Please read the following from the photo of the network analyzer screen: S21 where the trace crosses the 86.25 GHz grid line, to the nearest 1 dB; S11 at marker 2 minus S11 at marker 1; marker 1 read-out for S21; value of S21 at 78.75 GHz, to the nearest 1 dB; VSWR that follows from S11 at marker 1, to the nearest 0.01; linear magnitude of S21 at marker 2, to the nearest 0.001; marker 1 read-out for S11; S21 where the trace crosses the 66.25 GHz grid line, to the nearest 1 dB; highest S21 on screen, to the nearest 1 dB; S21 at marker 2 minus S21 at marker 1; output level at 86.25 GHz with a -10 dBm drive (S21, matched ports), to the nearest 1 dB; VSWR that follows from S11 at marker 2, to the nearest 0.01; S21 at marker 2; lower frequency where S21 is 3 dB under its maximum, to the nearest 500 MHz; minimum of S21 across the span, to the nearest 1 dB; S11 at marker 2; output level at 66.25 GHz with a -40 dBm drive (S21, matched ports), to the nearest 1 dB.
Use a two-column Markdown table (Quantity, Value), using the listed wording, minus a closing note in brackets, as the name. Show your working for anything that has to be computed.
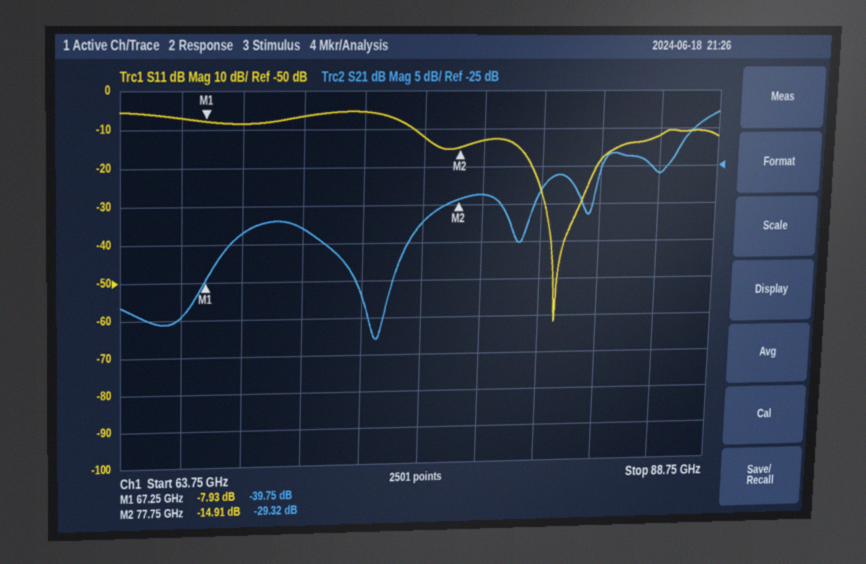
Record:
| Quantity | Value |
|---|---|
| S21 where the trace crosses the 86.25 GHz grid line, to the nearest 1 dB | -26 dB |
| S11 at marker 2 minus S11 at marker 1 | -14.91 − (-7.93) = -6.98 dB |
| marker 1 read-out for S21 | -39.75 dB |
| value of S21 at 78.75 GHz, to the nearest 1 dB | -29 dB |
| VSWR that follows from S11 at marker 1, to the nearest 0.01 | (1 + 0.4013)/(1 − 0.4013) ≈ 2.34 |
| linear magnitude of S21 at marker 2, to the nearest 0.001 | 10^(-29.32/20) ≈ 0.034 |
| marker 1 read-out for S11 | -7.93 dB |
| S21 where the trace crosses the 66.25 GHz grid line, to the nearest 1 dB | -45 dB |
| highest S21 on screen, to the nearest 1 dB | -18 dB |
| S21 at marker 2 minus S21 at marker 1 | -29.32 − (-39.75) = 10.43 dB |
| output level at 86.25 GHz with a -10 dBm drive (S21, matched ports), to the nearest 1 dB | -10 dBm + (-26 dB) = -36 dBm |
| VSWR that follows from S11 at marker 2, to the nearest 0.01 | (1 + 0.1797)/(1 − 0.1797) ≈ 1.44 |
| S21 at marker 2 | -29.32 dB |
| lower frequency where S21 is 3 dB under its maximum, to the nearest 500 MHz | 87.5 GHz |
| minimum of S21 across the span, to the nearest 1 dB | -48 dB |
| S11 at marker 2 | -14.91 dB |
| output level at 66.25 GHz with a -40 dBm drive (S21, matched ports), to the nearest 1 dB | -40 dBm + (-45 dB) = -85 dBm |
